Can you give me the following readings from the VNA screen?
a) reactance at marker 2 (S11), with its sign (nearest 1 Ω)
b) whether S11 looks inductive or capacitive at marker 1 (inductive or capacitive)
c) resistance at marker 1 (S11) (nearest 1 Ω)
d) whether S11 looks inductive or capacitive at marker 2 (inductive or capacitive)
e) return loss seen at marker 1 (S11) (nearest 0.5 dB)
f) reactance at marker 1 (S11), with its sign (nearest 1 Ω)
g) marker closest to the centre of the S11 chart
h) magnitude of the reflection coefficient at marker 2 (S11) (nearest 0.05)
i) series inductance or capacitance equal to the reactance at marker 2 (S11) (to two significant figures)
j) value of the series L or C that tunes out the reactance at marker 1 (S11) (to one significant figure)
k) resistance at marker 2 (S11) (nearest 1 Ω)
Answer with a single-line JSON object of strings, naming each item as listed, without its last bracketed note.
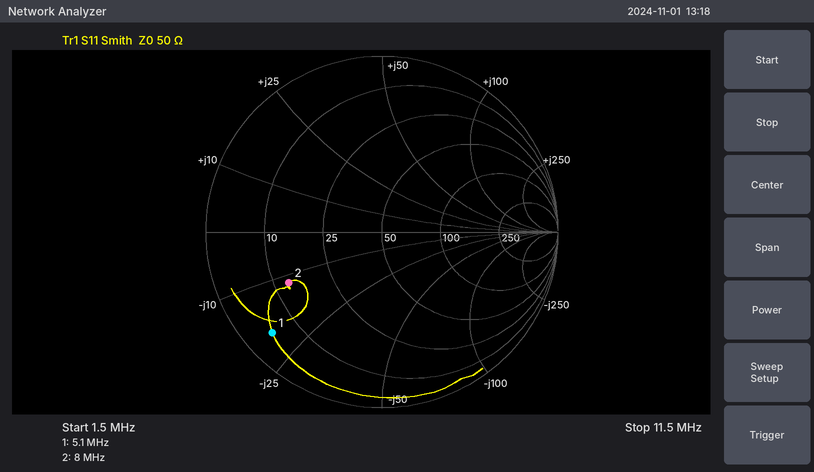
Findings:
{"reactance at marker 2 (S11), with its sign": "-12 Ω", "whether S11 looks inductive or capacitive at marker 1": "capacitive", "resistance at marker 1 (S11)": "5 Ω", "whether S11 looks inductive or capacitive at marker 2": "capacitive", "return loss seen at marker 1 (S11)": "1.5 dB", "reactance at marker 1 (S11), with its sign": "-19 Ω", "marker closest to the centre of the S11 chart": "marker 2", "magnitude of the reflection coefficient at marker 2 (S11)": "0.60", "series inductance or capacitance equal to the reactance at marker 2 (S11)": "1.7 nF", "value of the series L or C that tunes out the reactance at marker 1 (S11)": "600 nH", "resistance at marker 2 (S11)": "13 Ω"}
